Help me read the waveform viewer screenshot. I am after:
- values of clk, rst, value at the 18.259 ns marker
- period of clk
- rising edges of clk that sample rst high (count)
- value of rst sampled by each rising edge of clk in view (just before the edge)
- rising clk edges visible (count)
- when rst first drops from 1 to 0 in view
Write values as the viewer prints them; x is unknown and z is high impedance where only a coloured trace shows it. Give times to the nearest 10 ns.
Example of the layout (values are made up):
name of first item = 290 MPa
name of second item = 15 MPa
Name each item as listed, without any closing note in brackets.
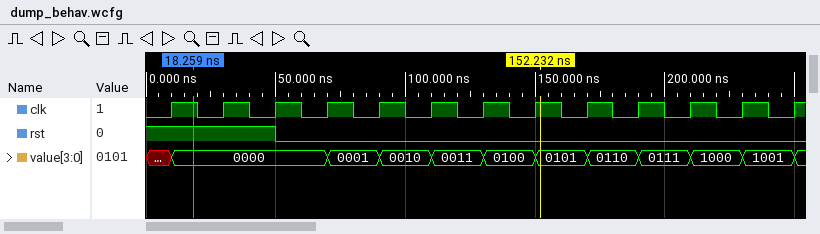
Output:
values of clk, rst, value at the 18.259 ns marker = clk=1, rst=1, value=0000
period of clk = 20 ns
rising edges of clk that sample rst high = 3
value of rst sampled by each rising edge of clk in view = 1 1 1 0 0 0 0 0 0 0 0 0 0
rising clk edges visible = 13
when rst first drops from 1 to 0 in view = 50 ns
